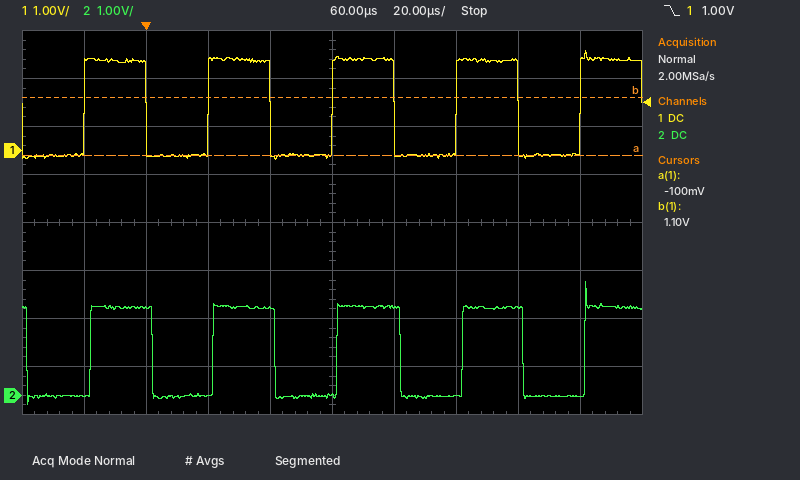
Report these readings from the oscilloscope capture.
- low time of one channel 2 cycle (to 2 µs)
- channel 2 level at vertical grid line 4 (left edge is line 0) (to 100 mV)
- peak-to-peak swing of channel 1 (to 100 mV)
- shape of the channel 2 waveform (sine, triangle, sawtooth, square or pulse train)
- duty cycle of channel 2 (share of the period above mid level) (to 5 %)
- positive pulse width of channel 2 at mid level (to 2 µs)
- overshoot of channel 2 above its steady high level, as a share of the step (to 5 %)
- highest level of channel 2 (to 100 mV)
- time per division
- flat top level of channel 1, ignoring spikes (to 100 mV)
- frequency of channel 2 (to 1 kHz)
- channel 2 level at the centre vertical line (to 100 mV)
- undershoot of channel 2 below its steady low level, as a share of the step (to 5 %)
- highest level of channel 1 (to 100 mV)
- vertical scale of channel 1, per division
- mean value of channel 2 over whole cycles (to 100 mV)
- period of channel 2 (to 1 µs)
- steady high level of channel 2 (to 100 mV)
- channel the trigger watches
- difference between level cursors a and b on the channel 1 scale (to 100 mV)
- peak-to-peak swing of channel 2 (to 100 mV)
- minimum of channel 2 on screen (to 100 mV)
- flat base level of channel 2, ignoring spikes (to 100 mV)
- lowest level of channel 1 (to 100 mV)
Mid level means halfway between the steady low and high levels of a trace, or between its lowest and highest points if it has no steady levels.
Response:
20 µs
1.8 V
2.3 V
square
50 %
20 µs
30 %
2.4 V
20 µs
1.9 V
25 kHz
0.0 V
10 %
2.1 V
1 V
900 mV
40 µs
1.8 V
channel 1
1.2 V
2.6 V
-200 mV
0.0 V
-200 mV
